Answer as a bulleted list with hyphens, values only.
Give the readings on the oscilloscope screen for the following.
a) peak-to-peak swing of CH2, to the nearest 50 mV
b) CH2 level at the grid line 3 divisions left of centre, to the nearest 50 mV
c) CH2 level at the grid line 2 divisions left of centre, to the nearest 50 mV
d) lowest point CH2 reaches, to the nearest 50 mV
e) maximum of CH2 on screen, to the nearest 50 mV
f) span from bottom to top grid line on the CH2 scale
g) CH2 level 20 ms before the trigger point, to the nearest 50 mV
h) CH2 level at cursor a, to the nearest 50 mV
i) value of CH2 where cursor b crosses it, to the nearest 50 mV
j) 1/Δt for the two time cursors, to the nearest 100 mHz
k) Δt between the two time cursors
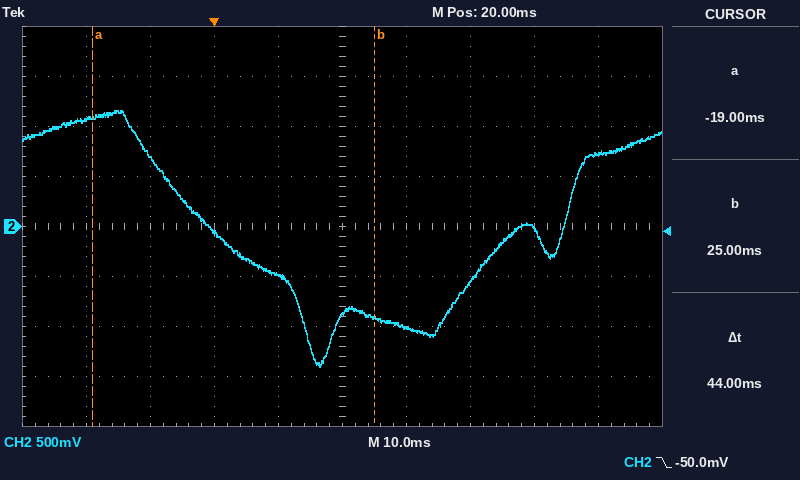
- 2.55 V
- 700 mV
- -50 mV
- -1.40 V
- 1.15 V
- 4 V
- 1.10 V
- 1.10 V
- -900 mV
- 22.7 Hz
- 44 ms
